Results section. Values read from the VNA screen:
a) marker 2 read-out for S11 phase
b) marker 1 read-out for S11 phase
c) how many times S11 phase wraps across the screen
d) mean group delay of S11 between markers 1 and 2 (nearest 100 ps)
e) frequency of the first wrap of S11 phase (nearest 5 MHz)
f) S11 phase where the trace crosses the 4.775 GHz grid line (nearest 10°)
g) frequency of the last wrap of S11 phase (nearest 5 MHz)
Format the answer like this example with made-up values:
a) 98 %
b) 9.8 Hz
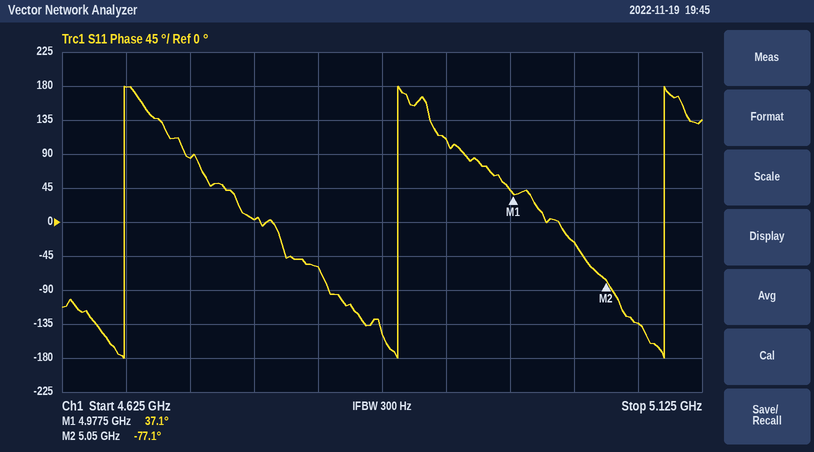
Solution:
a) -77.1°
b) 37.1°
c) 3
d) 4.4 ns
e) 4.675 GHz
f) 0°
g) 5.095 GHz
